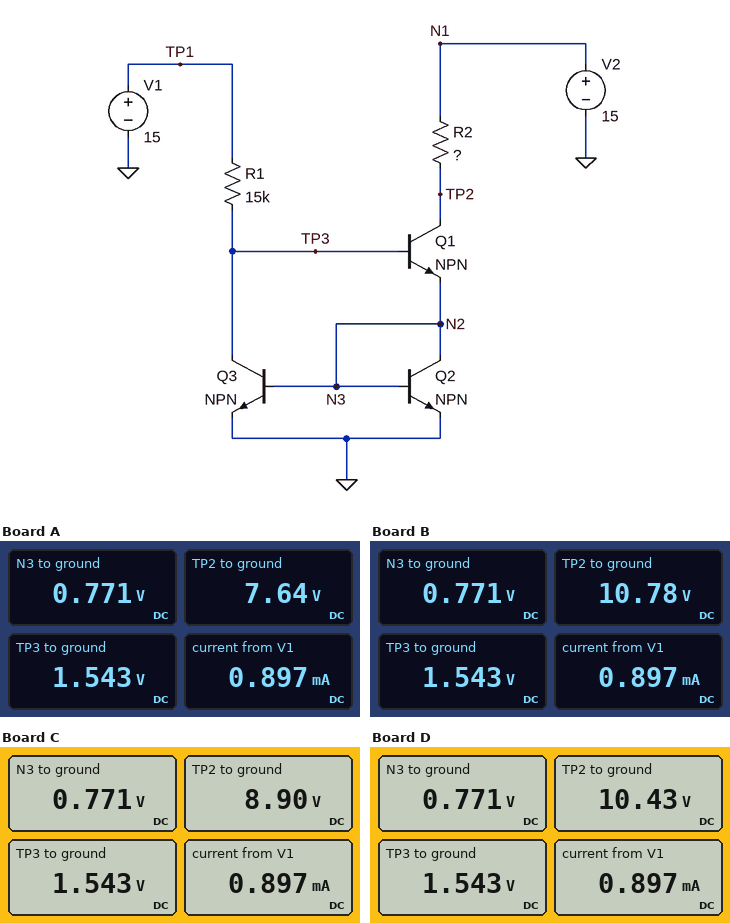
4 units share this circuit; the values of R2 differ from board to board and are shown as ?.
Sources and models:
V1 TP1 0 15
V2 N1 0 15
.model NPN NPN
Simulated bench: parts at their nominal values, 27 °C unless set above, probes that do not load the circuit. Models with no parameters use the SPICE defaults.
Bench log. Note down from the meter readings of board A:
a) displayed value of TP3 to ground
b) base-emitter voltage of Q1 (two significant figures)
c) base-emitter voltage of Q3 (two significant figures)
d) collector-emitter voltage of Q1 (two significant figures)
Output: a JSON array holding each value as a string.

["1.543 V", "770 mV", "770 mV", "6.9 V"]
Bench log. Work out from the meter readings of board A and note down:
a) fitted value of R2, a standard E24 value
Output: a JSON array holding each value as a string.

["8.2 kΩ"]
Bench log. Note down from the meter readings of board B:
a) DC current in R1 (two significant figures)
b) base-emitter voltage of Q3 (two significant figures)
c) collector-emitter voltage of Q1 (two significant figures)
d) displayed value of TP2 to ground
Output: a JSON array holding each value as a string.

["900 µA", "770 mV", "10 V", "10.78 V"]
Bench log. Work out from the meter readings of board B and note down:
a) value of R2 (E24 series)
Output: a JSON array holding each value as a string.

["4.7 kΩ"]
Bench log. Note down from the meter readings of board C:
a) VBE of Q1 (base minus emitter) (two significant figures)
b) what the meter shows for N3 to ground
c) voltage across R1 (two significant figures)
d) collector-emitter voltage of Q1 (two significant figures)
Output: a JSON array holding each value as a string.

["770 mV", "0.771 V", "13 V", "8.1 V"]
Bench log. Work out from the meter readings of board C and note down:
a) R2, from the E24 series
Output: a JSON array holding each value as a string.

["6.8 kΩ"]
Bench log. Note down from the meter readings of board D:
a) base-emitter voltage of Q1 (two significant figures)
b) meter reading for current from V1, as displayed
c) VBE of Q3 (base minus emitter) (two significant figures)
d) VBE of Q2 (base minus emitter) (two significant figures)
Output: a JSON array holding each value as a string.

["770 mV", "0.897 mA", "770 mV", "770 mV"]
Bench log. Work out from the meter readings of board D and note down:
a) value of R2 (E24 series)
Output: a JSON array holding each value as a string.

["5.1 kΩ"]
